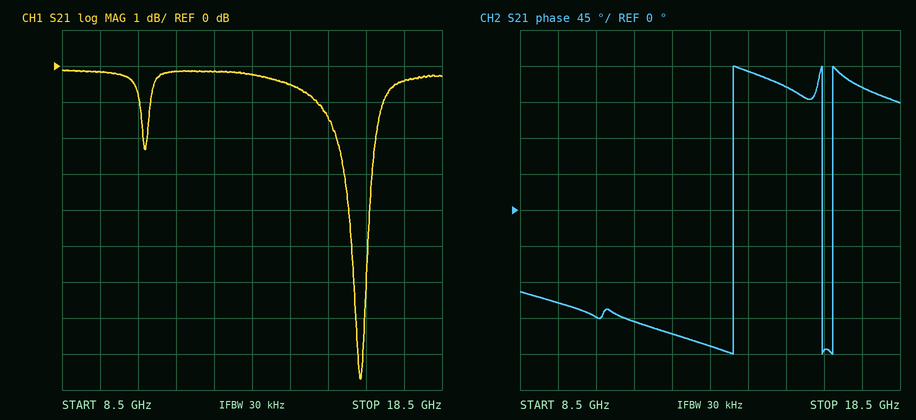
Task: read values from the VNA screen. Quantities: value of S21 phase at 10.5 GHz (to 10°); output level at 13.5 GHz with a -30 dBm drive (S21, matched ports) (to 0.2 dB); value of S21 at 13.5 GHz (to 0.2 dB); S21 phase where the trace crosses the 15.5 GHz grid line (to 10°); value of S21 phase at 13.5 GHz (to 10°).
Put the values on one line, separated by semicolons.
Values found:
-130°; -30.2 dBm; -0.2 dB; 150°; -170°
